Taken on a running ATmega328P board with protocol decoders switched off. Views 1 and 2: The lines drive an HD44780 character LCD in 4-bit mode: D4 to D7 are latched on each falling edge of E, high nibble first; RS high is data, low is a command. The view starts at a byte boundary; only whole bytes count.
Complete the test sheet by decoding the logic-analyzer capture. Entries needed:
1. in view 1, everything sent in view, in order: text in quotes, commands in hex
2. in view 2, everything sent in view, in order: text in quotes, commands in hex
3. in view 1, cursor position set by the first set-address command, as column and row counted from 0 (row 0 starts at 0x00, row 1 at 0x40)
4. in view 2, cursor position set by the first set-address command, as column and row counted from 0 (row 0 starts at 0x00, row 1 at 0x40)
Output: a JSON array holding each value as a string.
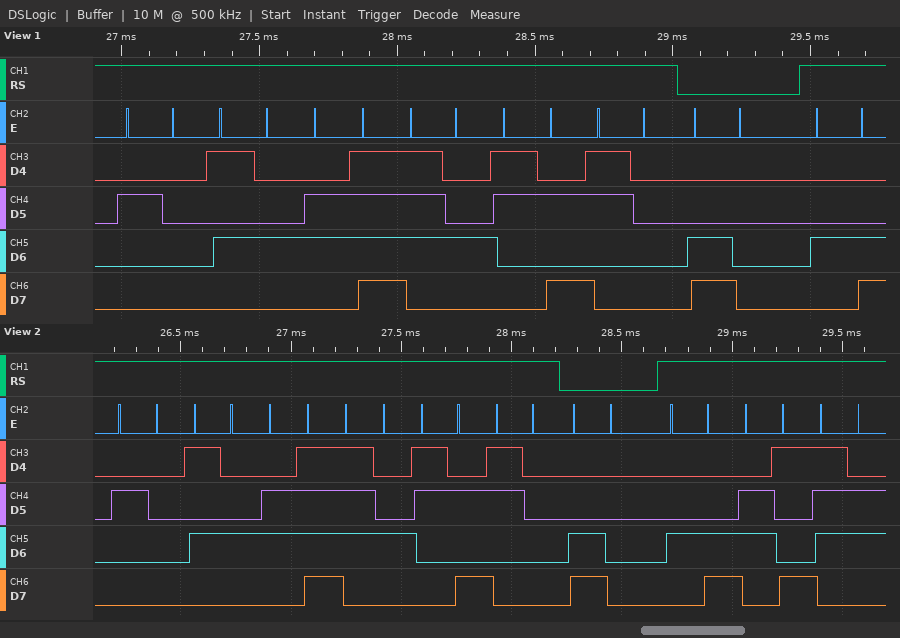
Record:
["\" Tot:0\" 0xC0 \"L\"", "\" Tot:0\" 0xC0 \"Liv\"", "column 0, row 1", "column 0, row 1"]
